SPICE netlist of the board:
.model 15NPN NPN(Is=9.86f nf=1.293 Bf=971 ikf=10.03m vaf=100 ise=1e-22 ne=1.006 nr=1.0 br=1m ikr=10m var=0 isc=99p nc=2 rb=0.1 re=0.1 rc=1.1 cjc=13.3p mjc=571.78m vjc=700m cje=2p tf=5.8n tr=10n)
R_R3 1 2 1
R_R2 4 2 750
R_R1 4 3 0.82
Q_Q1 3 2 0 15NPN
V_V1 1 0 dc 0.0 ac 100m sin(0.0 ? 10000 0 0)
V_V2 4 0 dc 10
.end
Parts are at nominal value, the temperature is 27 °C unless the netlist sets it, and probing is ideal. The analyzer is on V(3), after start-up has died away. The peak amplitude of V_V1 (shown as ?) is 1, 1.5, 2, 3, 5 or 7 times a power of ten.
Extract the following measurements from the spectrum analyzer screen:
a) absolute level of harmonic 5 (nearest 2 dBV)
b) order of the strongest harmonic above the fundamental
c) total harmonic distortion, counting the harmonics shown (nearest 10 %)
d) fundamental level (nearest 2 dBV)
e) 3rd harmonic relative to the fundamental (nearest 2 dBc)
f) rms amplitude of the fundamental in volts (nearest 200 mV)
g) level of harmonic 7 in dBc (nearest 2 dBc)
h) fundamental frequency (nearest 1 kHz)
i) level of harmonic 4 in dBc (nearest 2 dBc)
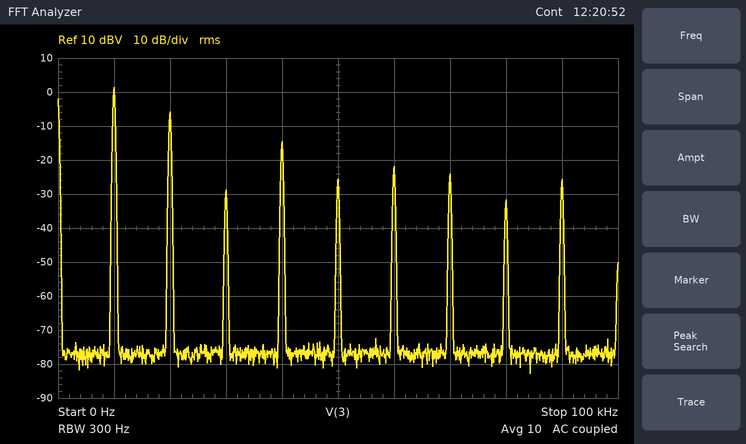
-26 dBV
2
50 %
2 dBV
-30 dBc
1.2 V
-26 dBc
10 kHz
-16 dBc
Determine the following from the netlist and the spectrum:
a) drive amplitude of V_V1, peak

5 V
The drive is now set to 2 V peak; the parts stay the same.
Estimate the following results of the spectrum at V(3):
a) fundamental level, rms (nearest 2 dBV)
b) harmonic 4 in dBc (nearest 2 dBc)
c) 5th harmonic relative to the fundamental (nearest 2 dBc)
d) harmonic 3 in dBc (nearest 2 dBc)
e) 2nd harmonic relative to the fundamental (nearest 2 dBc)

-8 dBV
-30 dBc
-20 dBc
-10 dBc
-4 dBc
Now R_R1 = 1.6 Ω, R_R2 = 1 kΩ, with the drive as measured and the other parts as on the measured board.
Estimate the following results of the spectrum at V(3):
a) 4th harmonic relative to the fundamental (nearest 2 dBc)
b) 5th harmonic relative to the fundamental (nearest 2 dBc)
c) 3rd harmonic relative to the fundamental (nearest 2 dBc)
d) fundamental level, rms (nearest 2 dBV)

-14 dBc
-24 dBc
-20 dBc
6 dBV
